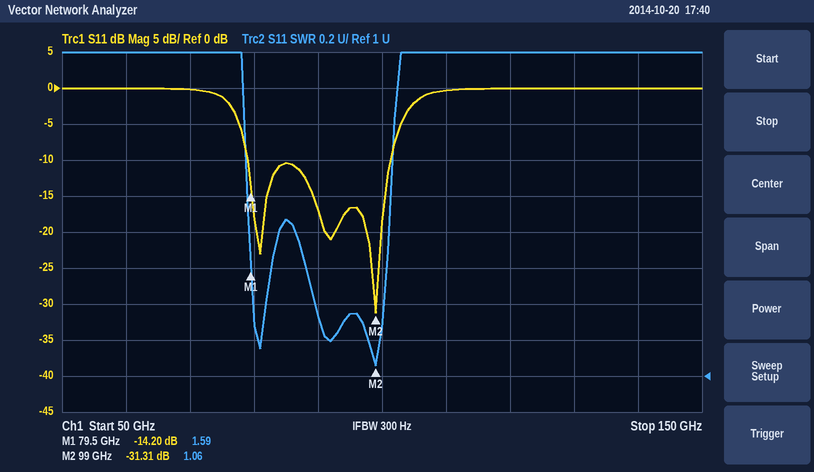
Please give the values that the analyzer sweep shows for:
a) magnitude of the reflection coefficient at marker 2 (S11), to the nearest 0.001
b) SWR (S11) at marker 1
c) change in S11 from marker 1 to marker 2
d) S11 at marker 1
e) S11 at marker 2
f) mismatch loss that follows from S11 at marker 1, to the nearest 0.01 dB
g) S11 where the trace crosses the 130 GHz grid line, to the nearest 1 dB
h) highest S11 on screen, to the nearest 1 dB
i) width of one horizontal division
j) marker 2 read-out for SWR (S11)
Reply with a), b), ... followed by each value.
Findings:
a) 0.027
b) 1.59
c) -17.11 dB
d) -14.20 dB
e) -31.31 dB
f) 0.17 dB
g) 0 dB
h) 0 dB
i) 10 GHz
j) 1.06
